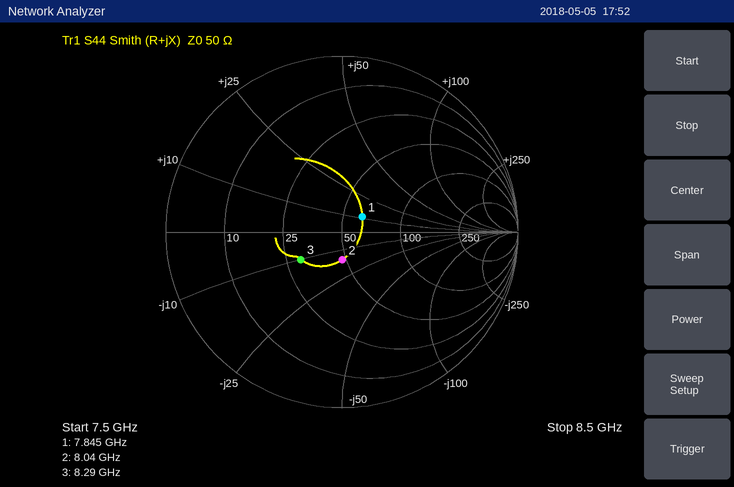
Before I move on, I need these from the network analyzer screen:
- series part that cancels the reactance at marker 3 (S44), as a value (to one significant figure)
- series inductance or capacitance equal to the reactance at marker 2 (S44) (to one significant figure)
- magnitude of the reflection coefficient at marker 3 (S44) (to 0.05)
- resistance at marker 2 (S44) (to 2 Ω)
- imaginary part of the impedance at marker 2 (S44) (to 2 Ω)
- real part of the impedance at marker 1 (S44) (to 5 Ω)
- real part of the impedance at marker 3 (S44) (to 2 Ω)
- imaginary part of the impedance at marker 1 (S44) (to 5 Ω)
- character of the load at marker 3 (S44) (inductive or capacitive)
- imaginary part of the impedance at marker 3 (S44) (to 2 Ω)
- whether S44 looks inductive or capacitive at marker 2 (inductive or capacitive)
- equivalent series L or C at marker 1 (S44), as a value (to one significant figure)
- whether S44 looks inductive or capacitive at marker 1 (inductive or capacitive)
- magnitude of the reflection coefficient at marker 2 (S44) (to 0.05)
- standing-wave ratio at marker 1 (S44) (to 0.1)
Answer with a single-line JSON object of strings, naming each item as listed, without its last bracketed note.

{"series part that cancels the reactance at marker 3 (S44), as a value": "200 pH", "series inductance or capacitance equal to the reactance at marker 2 (S44)": "1 pF", "magnitude of the reflection coefficient at marker 3 (S44)": "0.30", "resistance at marker 2 (S44)": "48 Ω", "imaginary part of the impedance at marker 2 (S44)": "-16 Ω", "real part of the impedance at marker 1 (S44)": "60 Ω", "real part of the impedance at marker 3 (S44)": "30 Ω", "imaginary part of the impedance at marker 1 (S44)": "+10 Ω", "character of the load at marker 3 (S44)": "capacitive", "imaginary part of the impedance at marker 3 (S44)": "-10 Ω", "whether S44 looks inductive or capacitive at marker 2": "capacitive", "equivalent series L or C at marker 1 (S44), as a value": "200 pH", "whether S44 looks inductive or capacitive at marker 1": "inductive", "magnitude of the reflection coefficient at marker 2 (S44)": "0.15", "standing-wave ratio at marker 1 (S44)": "1.3"}
